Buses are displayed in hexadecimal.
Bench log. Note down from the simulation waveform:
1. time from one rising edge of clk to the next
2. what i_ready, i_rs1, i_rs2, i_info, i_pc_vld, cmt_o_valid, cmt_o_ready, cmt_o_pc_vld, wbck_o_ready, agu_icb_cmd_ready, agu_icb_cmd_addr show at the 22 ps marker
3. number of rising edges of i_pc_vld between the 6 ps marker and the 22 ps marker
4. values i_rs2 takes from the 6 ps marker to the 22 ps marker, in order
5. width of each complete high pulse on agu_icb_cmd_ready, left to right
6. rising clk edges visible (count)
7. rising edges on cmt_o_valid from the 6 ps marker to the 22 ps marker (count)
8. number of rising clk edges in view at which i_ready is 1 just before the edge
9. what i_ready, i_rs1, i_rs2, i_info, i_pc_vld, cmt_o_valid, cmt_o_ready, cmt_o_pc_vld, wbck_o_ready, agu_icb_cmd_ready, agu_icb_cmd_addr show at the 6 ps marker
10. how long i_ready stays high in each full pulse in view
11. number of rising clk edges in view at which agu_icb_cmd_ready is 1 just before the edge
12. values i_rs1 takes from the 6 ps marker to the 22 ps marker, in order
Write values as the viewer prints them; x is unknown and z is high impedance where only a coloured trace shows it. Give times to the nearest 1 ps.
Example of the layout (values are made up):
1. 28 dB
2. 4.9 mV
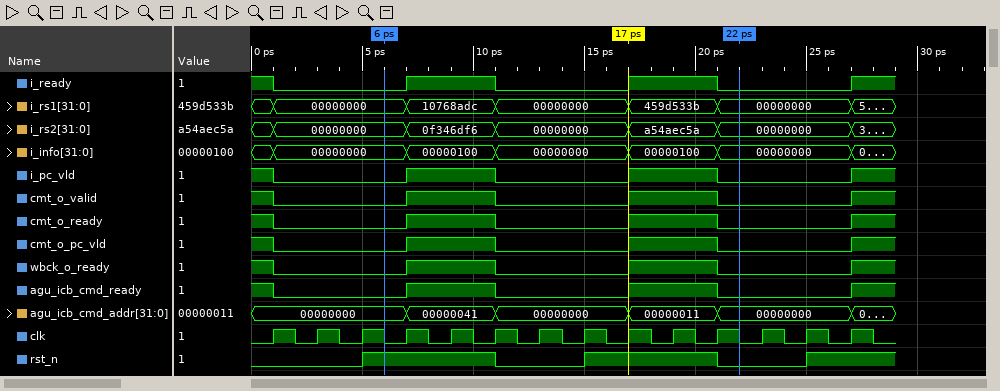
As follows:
1. 2 ps
2. i_ready=0, i_rs1=00000000, i_rs2=00000000, i_info=00000000, i_pc_vld=0, cmt_o_valid=0, cmt_o_ready=0, cmt_o_pc_vld=0, wbck_o_ready=0, agu_icb_cmd_ready=0, agu_icb_cmd_addr=00000000
3. 2
4. 00000000, 0f346df6, 00000000, a54aec5a, 00000000
5. 4 ps, 4 ps
6. 14
7. 2
8. 5
9. i_ready=0, i_rs1=00000000, i_rs2=00000000, i_info=00000000, i_pc_vld=0, cmt_o_valid=0, cmt_o_ready=0, cmt_o_pc_vld=0, wbck_o_ready=0, agu_icb_cmd_ready=0, agu_icb_cmd_addr=00000000
10. 4 ps, 4 ps
11. 5
12. 00000000, 10768adc, 00000000, 459d533b, 00000000
